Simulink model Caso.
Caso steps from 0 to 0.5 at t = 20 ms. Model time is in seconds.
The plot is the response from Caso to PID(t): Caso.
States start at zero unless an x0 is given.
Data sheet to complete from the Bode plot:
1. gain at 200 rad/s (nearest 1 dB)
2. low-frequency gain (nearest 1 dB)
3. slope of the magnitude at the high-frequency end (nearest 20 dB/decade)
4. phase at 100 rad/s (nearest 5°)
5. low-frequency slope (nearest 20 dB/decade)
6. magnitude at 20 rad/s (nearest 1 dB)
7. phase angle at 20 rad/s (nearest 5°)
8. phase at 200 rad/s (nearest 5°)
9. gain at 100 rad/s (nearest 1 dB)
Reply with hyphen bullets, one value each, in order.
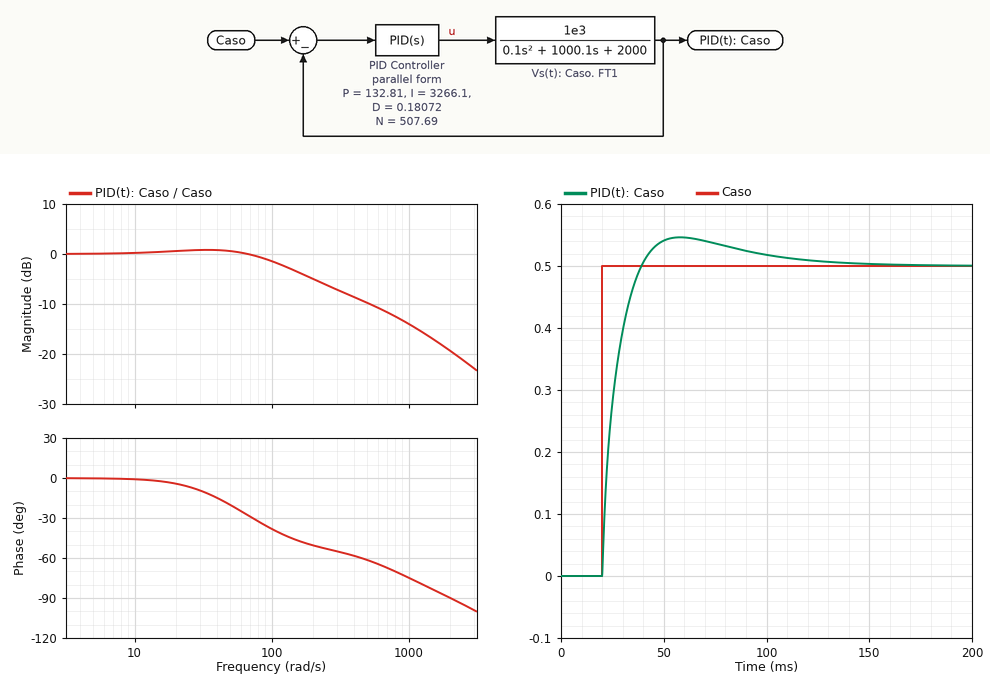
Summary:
- -5 dB
- 0 dB
- -20 dB/decade
- -40°
- 0 dB/decade
- 1 dB
- -5°
- -50°
- -1 dB
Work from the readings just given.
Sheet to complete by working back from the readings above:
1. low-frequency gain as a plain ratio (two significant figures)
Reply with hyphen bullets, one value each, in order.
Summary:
- 1.0
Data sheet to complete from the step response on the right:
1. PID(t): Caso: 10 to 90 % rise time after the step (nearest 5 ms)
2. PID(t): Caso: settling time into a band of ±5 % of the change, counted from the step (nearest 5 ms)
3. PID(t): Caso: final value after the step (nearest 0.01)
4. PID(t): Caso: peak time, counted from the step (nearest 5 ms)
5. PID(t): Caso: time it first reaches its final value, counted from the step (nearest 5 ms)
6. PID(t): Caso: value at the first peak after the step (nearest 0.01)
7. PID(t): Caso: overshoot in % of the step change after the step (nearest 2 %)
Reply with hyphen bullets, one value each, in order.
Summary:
- 15 ms
- 70 ms
- 0.50
- 40 ms
- 20 ms
- 0.55
- 10 %
